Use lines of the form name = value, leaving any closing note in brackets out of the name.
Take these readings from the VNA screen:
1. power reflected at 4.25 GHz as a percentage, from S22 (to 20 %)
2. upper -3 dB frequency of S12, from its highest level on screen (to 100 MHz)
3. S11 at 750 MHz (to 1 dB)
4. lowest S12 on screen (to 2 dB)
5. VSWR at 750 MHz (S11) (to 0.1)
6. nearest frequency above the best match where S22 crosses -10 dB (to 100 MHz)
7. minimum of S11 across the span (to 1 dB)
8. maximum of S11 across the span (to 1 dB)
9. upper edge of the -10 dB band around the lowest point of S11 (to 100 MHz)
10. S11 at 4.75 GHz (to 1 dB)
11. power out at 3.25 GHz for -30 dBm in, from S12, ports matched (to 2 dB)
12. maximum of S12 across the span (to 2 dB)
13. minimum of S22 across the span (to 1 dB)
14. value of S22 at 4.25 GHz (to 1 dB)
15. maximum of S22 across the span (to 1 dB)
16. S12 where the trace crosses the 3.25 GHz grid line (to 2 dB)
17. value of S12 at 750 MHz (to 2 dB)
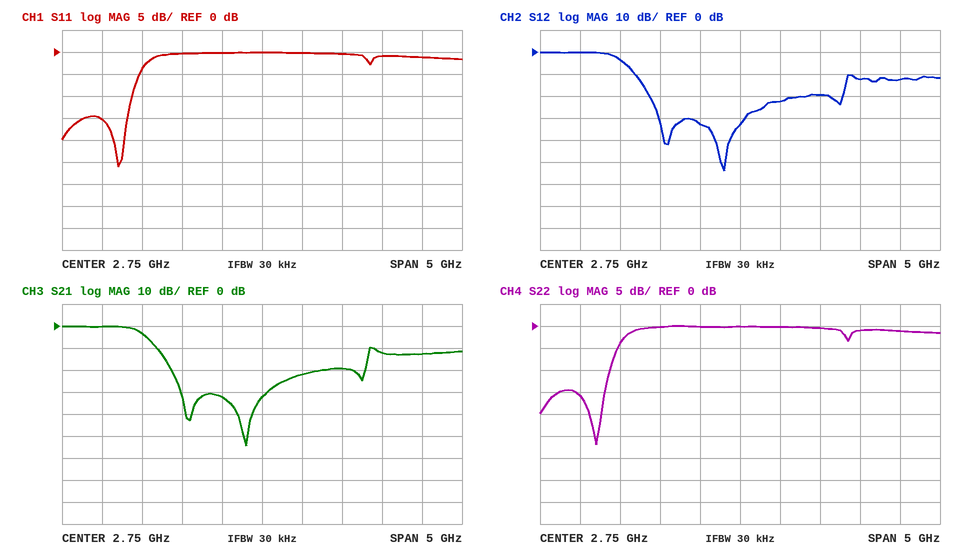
power reflected at 4.25 GHz as a percentage, from S22 = 80 %
upper -3 dB frequency of S12, from its highest level on screen = 1.2 GHz
S11 at 750 MHz = -15 dB
lowest S12 on screen = -54 dB
VSWR at 750 MHz (S11) = 1.4
nearest frequency above the best match where S22 crosses -10 dB = 1.1 GHz
minimum of S11 across the span = -26 dB
maximum of S11 across the span = 0 dB
upper edge of the -10 dB band around the lowest point of S11 = 1.1 GHz
S11 at 4.75 GHz = -1 dB
power out at 3.25 GHz for -30 dBm in, from S12, ports matched = -52 dBm
maximum of S12 across the span = 0 dB
minimum of S22 across the span = -27 dB
value of S22 at 4.25 GHz = -1 dB
maximum of S22 across the span = 0 dB
S12 where the trace crosses the 3.25 GHz grid line = -22 dB
value of S12 at 750 MHz = 0 dB
